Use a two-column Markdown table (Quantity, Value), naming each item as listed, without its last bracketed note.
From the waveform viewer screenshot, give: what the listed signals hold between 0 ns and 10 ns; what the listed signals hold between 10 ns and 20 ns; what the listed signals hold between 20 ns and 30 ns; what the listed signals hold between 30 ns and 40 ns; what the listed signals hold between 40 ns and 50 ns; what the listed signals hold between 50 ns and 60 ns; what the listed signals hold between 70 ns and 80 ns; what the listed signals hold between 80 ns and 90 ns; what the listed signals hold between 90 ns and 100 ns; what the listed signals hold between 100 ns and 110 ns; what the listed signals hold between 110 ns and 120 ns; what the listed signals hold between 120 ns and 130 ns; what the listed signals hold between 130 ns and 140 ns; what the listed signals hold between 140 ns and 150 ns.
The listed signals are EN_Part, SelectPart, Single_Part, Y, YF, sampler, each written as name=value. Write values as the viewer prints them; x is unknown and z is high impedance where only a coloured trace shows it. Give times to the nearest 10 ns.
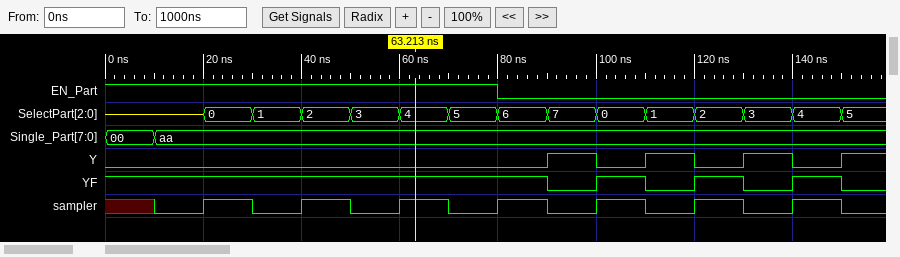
| Quantity | Value |
|---|---|
| what the listed signals hold between 0 ns and 10 ns | EN_Part=1, SelectPart=z, Single_Part=00, Y=0, YF=1, sampler=x |
| what the listed signals hold between 10 ns and 20 ns | EN_Part=1, SelectPart=z, Single_Part=aa, Y=0, YF=1, sampler=0 |
| what the listed signals hold between 20 ns and 30 ns | EN_Part=1, SelectPart=0, Single_Part=aa, Y=0, YF=1, sampler=1 |
| what the listed signals hold between 30 ns and 40 ns | EN_Part=1, SelectPart=1, Single_Part=aa, Y=0, YF=1, sampler=0 |
| what the listed signals hold between 40 ns and 50 ns | EN_Part=1, SelectPart=2, Single_Part=aa, Y=0, YF=1, sampler=1 |
| what the listed signals hold between 50 ns and 60 ns | EN_Part=1, SelectPart=3, Single_Part=aa, Y=0, YF=1, sampler=0 |
| what the listed signals hold between 70 ns and 80 ns | EN_Part=1, SelectPart=5, Single_Part=aa, Y=0, YF=1, sampler=0 |
| what the listed signals hold between 80 ns and 90 ns | EN_Part=0, SelectPart=6, Single_Part=aa, Y=0, YF=1, sampler=1 |
| what the listed signals hold between 90 ns and 100 ns | EN_Part=0, SelectPart=7, Single_Part=aa, Y=1, YF=0, sampler=0 |
| what the listed signals hold between 100 ns and 110 ns | EN_Part=0, SelectPart=0, Single_Part=aa, Y=0, YF=1, sampler=1 |
| what the listed signals hold between 110 ns and 120 ns | EN_Part=0, SelectPart=1, Single_Part=aa, Y=1, YF=0, sampler=0 |
| what the listed signals hold between 120 ns and 130 ns | EN_Part=0, SelectPart=2, Single_Part=aa, Y=0, YF=1, sampler=1 |
| what the listed signals hold between 130 ns and 140 ns | EN_Part=0, SelectPart=3, Single_Part=aa, Y=1, YF=0, sampler=0 |
| what the listed signals hold between 140 ns and 150 ns | EN_Part=0, SelectPart=4, Single_Part=aa, Y=0, YF=1, sampler=1 |
